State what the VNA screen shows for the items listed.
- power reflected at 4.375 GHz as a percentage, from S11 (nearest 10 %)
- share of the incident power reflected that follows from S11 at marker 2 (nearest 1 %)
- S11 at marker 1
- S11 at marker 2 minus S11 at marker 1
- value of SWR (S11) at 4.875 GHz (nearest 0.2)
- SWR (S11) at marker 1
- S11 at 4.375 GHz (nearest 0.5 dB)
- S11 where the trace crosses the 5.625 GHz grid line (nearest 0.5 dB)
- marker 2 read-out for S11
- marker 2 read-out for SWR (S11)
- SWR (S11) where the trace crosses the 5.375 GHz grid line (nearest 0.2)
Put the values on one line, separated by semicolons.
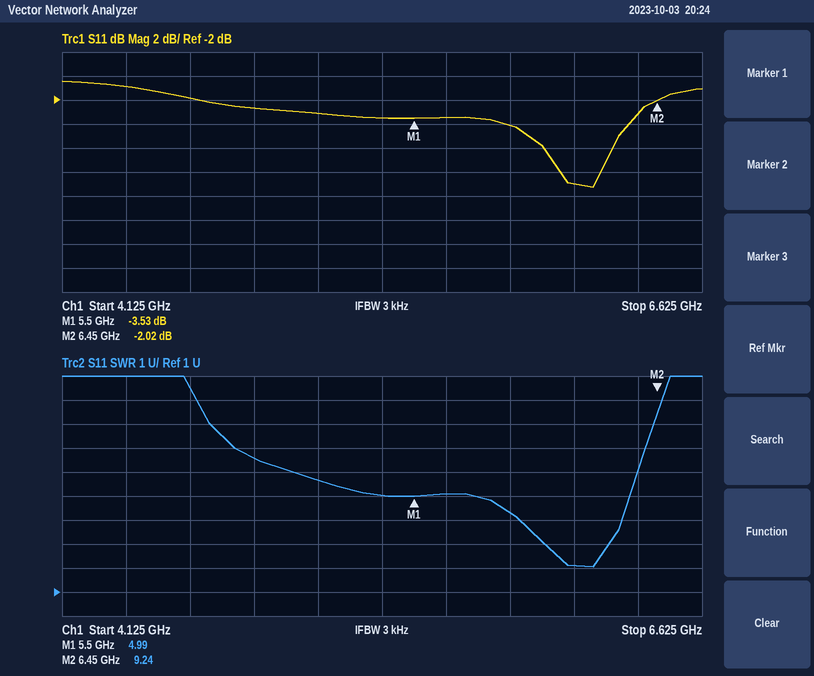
80 %; 63 %; -3.53 dB; 1.51 dB; 6.6; 4.99; -1.0 dB; -3.5 dB; -2.02 dB; 9.24; 5.0
